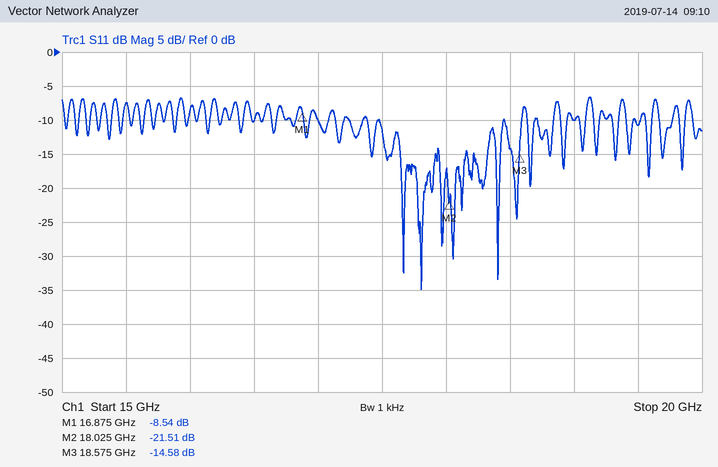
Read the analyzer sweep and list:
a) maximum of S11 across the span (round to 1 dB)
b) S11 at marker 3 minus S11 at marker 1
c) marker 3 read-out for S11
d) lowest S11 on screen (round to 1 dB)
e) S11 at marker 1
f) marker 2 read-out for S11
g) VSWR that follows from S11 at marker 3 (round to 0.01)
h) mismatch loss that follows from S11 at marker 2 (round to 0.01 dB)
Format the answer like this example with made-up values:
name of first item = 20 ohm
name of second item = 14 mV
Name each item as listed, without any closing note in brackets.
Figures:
maximum of S11 across the span = -7 dB
S11 at marker 3 minus S11 at marker 1 = -6.04 dB
marker 3 read-out for S11 = -14.58 dB
lowest S11 on screen = -35 dB
S11 at marker 1 = -8.54 dB
marker 2 read-out for S11 = -21.51 dB
VSWR that follows from S11 at marker 3 = 1.46
mismatch loss that follows from S11 at marker 2 = 0.03 dB
